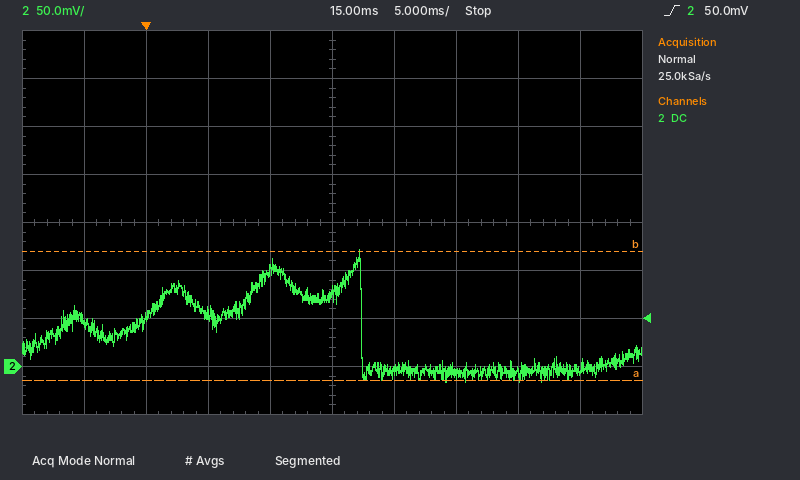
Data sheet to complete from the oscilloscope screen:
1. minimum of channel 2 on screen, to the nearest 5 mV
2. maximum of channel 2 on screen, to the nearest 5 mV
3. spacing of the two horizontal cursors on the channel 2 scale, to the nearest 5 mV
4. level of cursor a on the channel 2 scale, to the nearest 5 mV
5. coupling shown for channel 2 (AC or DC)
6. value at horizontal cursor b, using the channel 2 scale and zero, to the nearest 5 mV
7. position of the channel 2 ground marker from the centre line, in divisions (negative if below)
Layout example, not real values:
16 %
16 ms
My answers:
-15 mV
120 mV
135 mV
-15 mV
DC
120 mV
-3.0 div
